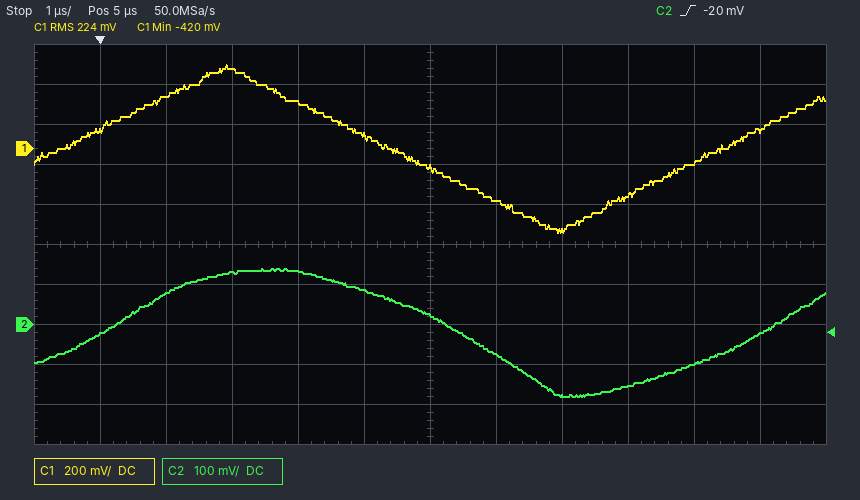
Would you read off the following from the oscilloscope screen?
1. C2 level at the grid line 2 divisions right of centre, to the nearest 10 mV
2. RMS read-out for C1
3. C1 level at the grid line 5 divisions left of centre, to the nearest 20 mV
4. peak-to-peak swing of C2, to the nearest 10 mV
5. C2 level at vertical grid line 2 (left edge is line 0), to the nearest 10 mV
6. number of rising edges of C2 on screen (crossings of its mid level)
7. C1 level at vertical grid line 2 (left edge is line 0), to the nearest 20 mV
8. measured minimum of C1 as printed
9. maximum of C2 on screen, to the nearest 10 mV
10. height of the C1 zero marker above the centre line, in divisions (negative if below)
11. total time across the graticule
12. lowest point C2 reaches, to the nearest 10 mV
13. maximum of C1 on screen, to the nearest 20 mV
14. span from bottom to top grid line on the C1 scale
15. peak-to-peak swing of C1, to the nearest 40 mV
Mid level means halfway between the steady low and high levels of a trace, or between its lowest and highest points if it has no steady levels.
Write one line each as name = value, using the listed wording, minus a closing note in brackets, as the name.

C2 level at the grid line 2 divisions right of centre, to the nearest 10 mV = -180 mV
RMS read-out for C1 = 224 mV
C1 level at the grid line 5 divisions left of centre, to the nearest 20 mV = 100 mV
peak-to-peak swing of C2, to the nearest 10 mV = 320 mV
C2 level at vertical grid line 2 (left edge is line 0), to the nearest 10 mV = 80 mV
number of rising edges of C2 on screen = 2
C1 level at vertical grid line 2 (left edge is line 0), to the nearest 20 mV = 260 mV
measured minimum of C1 as printed = -420 mV
maximum of C2 on screen, to the nearest 10 mV = 140 mV
height of the C1 zero marker above the centre line, in divisions = +2.4 div
total time across the graticule = 12 µs
lowest point C2 reaches, to the nearest 10 mV = -180 mV
maximum of C1 on screen, to the nearest 20 mV = 420 mV
span from bottom to top grid line on the C1 scale = 2 V
peak-to-peak swing of C1, to the nearest 40 mV = 840 mV
